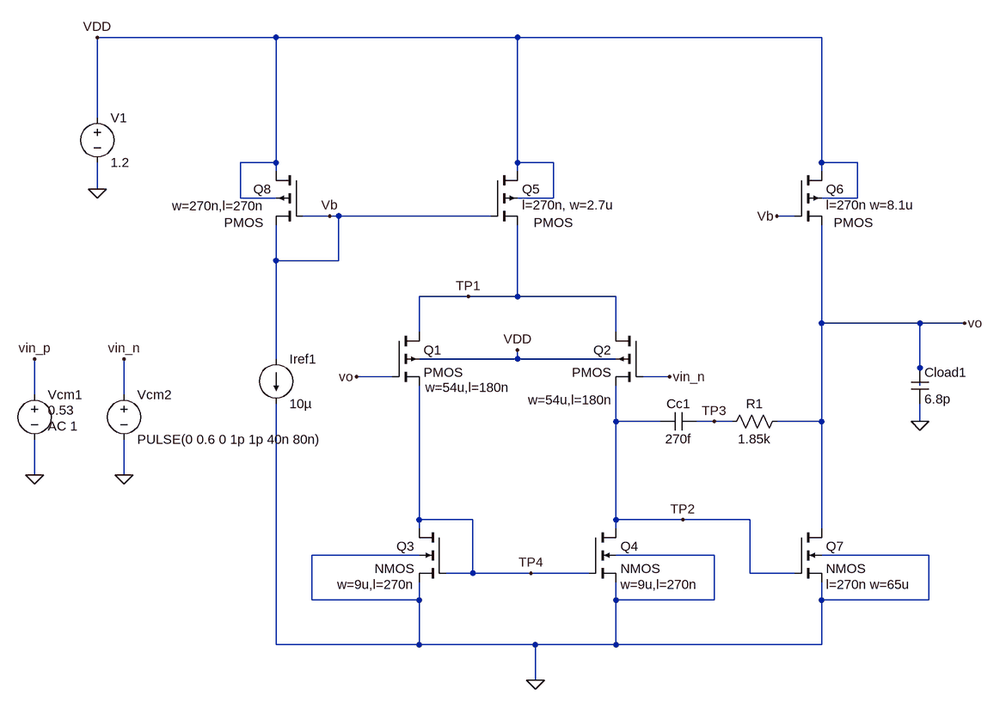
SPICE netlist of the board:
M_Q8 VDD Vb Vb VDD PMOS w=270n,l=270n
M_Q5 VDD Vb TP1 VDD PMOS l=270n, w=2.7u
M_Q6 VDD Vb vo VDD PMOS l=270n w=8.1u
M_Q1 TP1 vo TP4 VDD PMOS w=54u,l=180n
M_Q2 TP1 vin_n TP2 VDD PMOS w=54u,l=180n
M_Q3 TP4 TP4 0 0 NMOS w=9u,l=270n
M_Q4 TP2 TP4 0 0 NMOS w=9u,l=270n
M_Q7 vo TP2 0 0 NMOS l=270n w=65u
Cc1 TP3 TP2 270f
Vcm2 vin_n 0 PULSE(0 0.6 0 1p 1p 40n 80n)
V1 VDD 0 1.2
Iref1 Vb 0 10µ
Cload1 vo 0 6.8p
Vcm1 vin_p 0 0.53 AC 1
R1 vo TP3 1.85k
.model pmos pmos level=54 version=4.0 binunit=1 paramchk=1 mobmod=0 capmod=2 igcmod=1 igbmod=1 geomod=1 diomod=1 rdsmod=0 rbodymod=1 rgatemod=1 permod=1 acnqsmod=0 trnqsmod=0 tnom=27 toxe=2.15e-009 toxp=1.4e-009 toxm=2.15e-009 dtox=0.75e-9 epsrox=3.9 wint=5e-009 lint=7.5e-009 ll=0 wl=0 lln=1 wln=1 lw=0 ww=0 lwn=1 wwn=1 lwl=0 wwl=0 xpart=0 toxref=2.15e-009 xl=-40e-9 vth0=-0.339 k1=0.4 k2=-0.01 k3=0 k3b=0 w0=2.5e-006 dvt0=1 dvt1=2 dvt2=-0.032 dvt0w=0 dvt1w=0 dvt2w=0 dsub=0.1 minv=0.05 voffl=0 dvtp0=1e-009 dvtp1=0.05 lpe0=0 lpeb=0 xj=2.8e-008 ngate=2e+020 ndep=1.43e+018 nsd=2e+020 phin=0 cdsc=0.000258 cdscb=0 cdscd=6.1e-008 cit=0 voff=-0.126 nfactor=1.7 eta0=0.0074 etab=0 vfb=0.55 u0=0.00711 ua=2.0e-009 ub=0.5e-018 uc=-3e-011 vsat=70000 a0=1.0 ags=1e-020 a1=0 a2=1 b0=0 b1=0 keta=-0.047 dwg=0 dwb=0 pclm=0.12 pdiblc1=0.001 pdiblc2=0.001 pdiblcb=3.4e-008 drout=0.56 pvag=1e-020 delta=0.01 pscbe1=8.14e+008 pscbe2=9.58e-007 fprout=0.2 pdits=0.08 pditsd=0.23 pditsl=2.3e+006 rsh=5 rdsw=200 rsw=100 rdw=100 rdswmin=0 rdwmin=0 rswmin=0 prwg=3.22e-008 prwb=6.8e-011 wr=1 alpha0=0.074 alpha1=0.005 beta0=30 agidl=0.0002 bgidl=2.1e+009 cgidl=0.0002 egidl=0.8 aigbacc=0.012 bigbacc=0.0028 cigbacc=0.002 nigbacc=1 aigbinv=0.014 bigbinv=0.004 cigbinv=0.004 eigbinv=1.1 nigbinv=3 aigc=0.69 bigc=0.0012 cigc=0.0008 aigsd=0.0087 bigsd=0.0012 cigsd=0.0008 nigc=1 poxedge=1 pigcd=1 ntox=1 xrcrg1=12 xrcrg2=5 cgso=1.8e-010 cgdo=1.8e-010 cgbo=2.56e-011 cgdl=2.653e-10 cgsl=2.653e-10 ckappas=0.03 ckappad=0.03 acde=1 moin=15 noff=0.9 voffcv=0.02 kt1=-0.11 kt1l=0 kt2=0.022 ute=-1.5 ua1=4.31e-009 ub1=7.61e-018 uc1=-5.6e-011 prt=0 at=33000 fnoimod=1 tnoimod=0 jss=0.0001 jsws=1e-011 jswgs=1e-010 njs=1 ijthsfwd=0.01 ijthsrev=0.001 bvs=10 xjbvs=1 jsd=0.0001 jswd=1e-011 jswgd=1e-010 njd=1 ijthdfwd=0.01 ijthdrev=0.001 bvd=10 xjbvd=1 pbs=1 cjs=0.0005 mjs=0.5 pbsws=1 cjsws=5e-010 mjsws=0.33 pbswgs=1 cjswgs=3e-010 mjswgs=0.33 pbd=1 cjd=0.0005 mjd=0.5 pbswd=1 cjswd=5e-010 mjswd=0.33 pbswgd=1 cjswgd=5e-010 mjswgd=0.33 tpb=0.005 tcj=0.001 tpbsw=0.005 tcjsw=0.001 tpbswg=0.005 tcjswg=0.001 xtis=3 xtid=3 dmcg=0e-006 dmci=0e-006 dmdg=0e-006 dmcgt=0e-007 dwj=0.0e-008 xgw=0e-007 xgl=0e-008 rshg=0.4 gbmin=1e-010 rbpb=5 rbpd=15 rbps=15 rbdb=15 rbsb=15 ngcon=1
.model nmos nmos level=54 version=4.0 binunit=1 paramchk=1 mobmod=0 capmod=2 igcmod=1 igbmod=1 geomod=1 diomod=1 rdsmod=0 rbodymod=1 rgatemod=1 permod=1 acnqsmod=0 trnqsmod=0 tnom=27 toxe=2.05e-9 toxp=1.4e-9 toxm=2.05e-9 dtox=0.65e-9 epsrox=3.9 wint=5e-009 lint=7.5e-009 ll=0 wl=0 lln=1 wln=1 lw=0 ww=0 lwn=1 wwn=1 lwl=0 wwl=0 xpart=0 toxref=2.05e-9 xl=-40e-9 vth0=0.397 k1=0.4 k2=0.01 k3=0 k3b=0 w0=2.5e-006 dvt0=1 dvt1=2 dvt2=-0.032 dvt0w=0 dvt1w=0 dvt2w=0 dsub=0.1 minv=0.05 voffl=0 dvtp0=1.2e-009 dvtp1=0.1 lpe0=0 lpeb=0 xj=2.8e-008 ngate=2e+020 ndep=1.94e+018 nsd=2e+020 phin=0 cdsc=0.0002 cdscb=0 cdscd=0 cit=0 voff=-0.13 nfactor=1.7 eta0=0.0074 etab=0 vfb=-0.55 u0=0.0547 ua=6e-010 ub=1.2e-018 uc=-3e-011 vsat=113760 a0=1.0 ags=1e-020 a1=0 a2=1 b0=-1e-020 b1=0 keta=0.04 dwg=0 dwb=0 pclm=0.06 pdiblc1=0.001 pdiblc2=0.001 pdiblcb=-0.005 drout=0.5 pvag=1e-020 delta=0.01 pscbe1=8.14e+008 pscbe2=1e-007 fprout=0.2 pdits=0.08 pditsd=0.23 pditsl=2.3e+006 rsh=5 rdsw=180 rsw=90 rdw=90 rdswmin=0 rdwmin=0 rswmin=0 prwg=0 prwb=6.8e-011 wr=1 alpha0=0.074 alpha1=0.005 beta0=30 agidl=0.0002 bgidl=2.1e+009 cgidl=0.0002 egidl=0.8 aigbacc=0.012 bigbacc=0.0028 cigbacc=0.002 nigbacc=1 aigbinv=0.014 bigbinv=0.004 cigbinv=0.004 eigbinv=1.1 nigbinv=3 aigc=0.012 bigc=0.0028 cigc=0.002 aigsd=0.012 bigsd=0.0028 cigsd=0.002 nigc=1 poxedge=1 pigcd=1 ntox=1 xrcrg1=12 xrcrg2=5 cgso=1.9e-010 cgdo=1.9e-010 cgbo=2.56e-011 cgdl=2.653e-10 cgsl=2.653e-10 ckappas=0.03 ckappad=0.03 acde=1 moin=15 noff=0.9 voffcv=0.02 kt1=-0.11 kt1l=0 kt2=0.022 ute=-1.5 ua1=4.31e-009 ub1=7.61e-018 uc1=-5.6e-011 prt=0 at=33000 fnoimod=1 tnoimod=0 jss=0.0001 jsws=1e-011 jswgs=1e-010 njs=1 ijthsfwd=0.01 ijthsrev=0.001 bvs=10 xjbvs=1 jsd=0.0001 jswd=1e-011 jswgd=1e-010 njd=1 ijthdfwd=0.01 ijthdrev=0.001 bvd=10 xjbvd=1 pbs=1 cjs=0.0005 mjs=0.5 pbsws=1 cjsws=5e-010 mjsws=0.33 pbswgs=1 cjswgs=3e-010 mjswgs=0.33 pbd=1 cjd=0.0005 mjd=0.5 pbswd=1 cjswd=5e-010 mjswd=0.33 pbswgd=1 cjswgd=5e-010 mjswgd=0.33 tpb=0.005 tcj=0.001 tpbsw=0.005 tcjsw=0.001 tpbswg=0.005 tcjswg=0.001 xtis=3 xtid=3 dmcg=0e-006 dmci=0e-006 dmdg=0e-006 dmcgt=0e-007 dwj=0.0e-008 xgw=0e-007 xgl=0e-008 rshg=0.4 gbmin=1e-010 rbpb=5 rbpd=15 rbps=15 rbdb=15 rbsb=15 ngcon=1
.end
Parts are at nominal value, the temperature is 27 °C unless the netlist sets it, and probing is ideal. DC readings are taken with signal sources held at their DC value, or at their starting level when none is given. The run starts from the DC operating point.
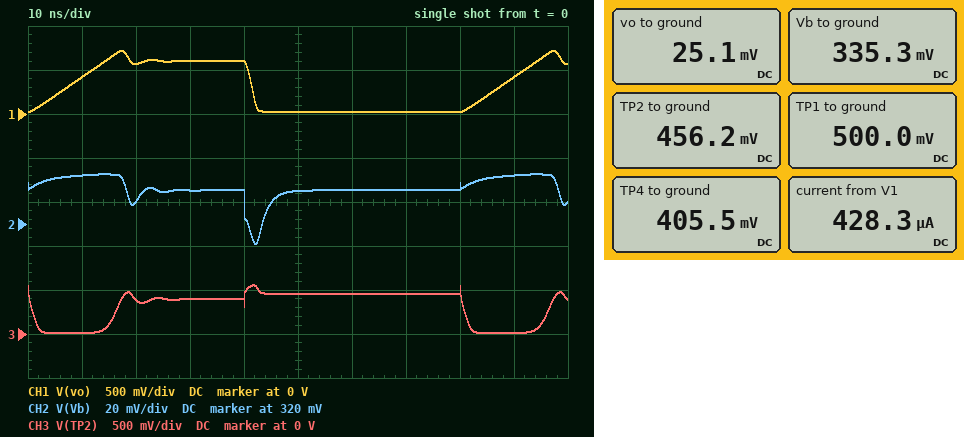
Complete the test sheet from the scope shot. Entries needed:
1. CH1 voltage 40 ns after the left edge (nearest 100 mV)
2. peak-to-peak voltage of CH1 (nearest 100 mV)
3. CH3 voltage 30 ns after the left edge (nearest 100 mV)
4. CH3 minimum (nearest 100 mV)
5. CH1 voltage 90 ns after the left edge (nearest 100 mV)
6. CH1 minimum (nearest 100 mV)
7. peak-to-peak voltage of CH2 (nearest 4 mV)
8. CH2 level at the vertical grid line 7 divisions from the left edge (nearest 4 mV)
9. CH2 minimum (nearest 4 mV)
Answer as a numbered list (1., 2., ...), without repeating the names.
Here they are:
1. 600 mV
2. 700 mV
3. 400 mV
4. 0 V
5. 400 mV
6. 0 V
7. 32 mV
8. 336 mV
9. 312 mV
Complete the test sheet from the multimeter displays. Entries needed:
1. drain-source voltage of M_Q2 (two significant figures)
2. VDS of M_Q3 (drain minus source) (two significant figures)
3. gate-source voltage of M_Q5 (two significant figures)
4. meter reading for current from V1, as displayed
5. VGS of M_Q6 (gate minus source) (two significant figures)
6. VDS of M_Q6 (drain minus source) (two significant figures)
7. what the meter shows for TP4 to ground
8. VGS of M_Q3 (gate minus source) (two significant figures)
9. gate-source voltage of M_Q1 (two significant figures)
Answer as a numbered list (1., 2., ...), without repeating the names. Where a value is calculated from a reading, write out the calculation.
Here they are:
1. 500 mV - 456.2 mV = 44 mV
2. 405.5 mV = 410 mV
3. 335.3 mV - 500 mV = -160 mV
4. 428.3 µA
5. 335.3 mV - 25.1 mV = 310 mV
6. 1.2 V - 25.1 mV = 1.2 V
7. 405.5 mV
8. 405.5 mV = 410 mV
9. 25.1 mV - 405.5 mV = -380 mV
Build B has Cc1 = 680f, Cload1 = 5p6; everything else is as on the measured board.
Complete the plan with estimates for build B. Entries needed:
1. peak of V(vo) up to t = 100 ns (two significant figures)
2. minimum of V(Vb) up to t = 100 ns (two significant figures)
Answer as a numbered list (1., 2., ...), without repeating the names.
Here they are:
1. 730 mV
2. 320 mV
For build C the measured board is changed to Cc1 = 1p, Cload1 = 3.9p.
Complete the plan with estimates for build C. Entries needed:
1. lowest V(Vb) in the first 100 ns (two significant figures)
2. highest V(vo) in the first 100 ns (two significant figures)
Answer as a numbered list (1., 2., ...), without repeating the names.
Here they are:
1. 320 mV
2. 680 mV
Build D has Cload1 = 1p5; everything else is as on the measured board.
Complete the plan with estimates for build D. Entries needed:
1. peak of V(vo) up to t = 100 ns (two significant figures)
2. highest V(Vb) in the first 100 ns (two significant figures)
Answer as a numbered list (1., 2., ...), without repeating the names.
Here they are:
1. 790 mV
2. 360 mV
